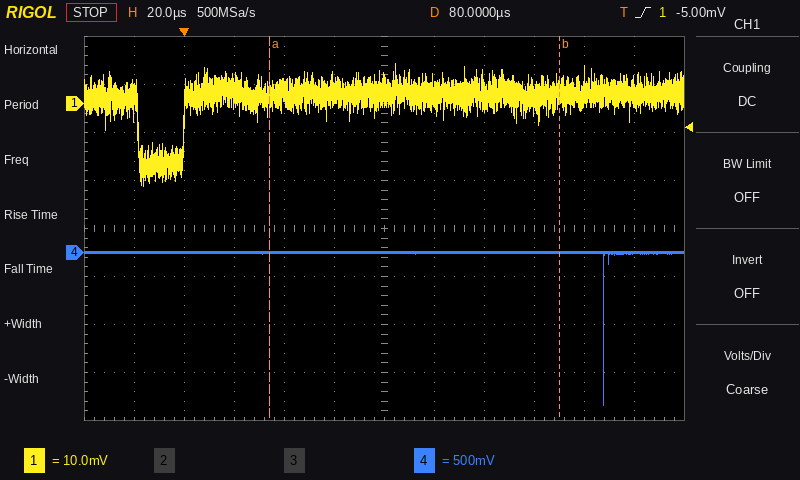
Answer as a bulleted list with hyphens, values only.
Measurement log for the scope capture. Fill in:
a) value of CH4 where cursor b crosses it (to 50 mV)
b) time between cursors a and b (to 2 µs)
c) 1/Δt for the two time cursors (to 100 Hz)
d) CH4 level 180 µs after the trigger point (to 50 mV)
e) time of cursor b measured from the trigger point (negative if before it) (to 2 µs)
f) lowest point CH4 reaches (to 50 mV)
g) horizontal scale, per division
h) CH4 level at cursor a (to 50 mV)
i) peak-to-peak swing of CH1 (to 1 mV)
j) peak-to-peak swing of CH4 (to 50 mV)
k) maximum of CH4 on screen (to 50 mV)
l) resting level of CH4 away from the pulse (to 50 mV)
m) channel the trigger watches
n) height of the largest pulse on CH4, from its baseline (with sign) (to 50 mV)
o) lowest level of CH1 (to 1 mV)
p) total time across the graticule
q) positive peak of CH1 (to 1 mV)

- 0 mV
- 116 µs
- 8.6 kHz
- 0 mV
- +150 µs
- -1.60 V
- 20 µs
- 0 mV
- 25 mV
- 1.60 V
- 0 mV
- 0 mV
- CH1
- -1.60 V
- -17 mV
- 240 µs
- 8 mV
